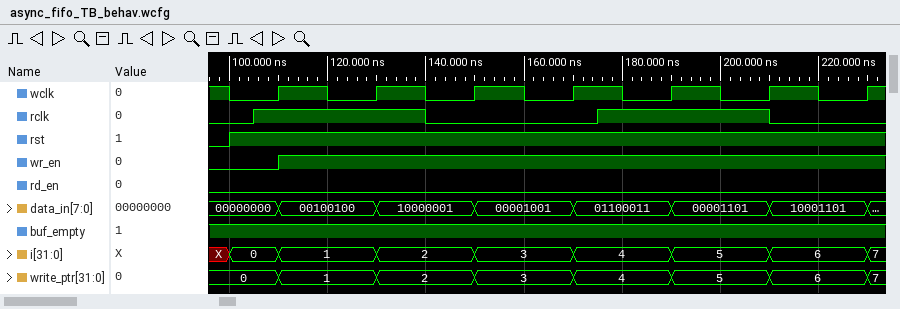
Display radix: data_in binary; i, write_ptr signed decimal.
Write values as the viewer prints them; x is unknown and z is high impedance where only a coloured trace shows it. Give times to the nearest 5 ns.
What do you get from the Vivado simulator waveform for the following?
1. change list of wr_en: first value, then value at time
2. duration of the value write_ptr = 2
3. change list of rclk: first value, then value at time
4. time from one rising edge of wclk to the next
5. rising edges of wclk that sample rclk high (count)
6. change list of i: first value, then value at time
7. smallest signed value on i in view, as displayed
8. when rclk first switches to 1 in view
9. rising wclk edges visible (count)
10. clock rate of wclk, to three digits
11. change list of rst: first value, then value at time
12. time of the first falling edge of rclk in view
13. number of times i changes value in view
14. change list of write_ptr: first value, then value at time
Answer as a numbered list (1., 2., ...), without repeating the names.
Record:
1. 0, 1 at 110 ns
2. 20 ns
3. 0, 1 at 105 ns, 0 at 140 ns, 1 at 175 ns, 0 at 210 ns
4. 20 ns
5. 4
6. X, 0 at 100 ns, 1 at 110 ns, 2 at 130 ns, 3 at 150 ns, 4 at 170 ns, 5 at 190 ns, 6 at 210 ns, 7 at 230 ns
7. 0
8. 105 ns
9. 7
10. 50.0 MHz
11. 0, 1 at 100 ns
12. 140 ns
13. 8
14. 0, 1 at 110 ns, 2 at 130 ns, 3 at 150 ns, 4 at 170 ns, 5 at 190 ns, 6 at 210 ns, 7 at 230 ns
